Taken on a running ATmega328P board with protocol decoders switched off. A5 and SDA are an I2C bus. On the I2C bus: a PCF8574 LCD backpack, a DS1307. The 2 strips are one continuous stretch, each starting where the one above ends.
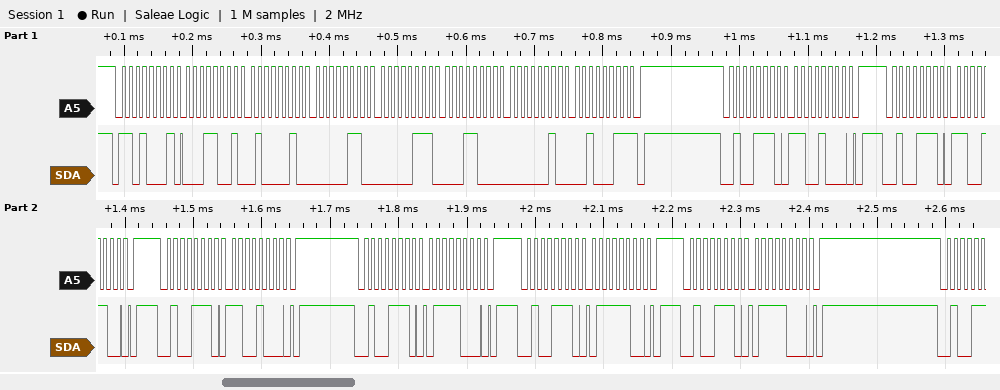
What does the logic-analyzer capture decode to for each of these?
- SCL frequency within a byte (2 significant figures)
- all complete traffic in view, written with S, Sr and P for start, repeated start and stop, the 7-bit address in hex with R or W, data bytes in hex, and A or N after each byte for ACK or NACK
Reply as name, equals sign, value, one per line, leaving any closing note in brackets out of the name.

SCL frequency within a byte = 100 kHz
all complete traffic in view, written with S, Sr and P for start, repeated start and stop, the 7-bit address in hex with R or W, data bytes in hex, and A or N after each byte for ACK or NACK = S 68R A 19 A 42 A 06 A 07 A 18 A 02 A 23 N P S 27W A C8 A P S 27W A CC A P S 27W A C8 A P S 27W A 78 A P S 27W A 7C A P S 27W A 78 A P
